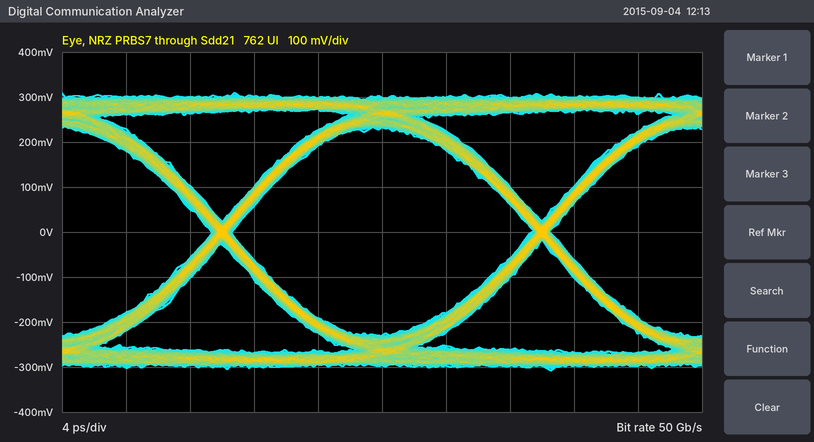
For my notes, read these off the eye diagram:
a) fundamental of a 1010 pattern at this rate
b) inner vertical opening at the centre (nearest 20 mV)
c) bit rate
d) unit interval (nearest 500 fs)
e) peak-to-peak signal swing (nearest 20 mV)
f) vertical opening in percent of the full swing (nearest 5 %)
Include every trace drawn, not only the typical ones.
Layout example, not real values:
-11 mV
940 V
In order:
25 GHz
460 mV
50 Gb/s
20.0 ps
620 mV
75 %
